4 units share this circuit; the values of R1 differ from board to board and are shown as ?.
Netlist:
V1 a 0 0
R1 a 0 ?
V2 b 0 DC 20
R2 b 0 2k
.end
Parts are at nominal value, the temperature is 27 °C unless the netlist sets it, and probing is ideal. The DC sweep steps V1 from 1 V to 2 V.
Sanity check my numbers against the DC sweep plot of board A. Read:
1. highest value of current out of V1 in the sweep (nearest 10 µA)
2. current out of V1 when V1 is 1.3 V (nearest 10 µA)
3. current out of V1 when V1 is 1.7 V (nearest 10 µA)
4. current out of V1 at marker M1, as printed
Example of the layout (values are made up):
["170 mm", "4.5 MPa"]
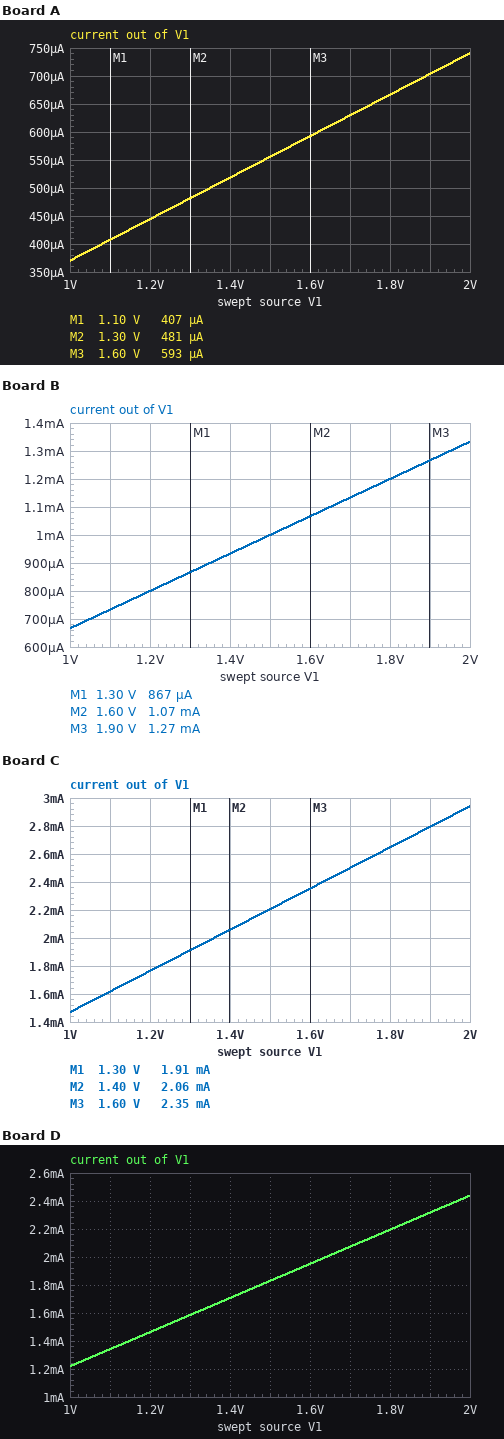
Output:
["740 µA", "480 µA", "630 µA", "407 µA"]
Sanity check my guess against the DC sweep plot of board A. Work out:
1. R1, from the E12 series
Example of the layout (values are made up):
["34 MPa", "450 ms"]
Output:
["2.7 kΩ"]
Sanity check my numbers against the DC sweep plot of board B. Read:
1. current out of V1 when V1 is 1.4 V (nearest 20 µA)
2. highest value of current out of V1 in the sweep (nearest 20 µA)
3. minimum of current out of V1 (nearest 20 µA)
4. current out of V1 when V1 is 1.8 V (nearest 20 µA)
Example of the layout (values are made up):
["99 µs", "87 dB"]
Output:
["940 µA", "1.34 mA", "660 µA", "1.20 mA"]
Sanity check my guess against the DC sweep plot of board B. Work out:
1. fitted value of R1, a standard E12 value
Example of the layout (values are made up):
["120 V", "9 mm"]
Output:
["1.5 kΩ"]
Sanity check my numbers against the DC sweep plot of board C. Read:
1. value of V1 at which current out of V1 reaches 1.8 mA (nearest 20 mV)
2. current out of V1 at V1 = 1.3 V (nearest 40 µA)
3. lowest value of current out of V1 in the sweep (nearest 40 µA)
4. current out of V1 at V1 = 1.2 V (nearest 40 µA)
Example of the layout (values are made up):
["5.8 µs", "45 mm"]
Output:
["1.22 V", "1.92 mA", "1.48 mA", "1.76 mA"]
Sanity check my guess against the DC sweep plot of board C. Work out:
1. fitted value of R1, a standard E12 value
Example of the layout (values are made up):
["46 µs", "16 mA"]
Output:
["680 Ω"]
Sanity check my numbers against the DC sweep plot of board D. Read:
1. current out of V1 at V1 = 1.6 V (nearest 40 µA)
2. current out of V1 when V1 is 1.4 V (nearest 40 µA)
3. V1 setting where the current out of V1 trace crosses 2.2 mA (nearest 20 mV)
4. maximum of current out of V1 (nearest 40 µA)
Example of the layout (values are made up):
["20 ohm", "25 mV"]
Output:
["1.96 mA", "1.72 mA", "1.80 V", "2.44 mA"]
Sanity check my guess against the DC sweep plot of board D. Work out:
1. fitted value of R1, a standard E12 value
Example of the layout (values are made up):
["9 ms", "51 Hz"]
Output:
["820 Ω"]
